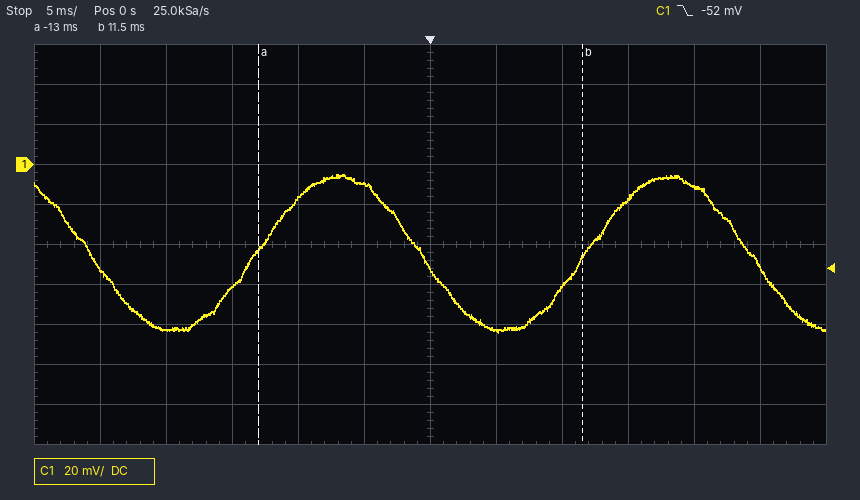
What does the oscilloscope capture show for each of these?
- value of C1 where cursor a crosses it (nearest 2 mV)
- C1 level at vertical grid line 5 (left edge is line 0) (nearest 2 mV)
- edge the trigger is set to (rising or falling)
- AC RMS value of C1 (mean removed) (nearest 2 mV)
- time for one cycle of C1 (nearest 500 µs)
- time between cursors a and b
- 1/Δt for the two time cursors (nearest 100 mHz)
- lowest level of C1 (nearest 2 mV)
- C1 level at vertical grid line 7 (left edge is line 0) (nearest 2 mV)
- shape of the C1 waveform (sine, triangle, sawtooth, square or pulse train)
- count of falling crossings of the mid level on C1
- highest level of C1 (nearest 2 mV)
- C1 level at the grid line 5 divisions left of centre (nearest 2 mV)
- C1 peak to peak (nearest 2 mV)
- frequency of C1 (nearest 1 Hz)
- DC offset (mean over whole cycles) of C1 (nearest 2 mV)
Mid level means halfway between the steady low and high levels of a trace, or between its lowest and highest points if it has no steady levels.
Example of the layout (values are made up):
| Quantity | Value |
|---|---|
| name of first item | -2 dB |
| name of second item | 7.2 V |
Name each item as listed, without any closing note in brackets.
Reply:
| Quantity | Value |
|---|---|
| value of C1 where cursor a crosses it | -42 mV |
| C1 level at vertical grid line 5 (left edge is line 0) | -10 mV |
| edge the trigger is set to | falling |
| AC RMS value of C1 (mean removed) | 28 mV |
| time for one cycle of C1 | 25.0 ms |
| time between cursors a and b | 24.5 ms |
| 1/Δt for the two time cursors | 40.8 Hz |
| lowest level of C1 | -84 mV |
| C1 level at vertical grid line 7 (left edge is line 0) | -84 mV |
| shape of the C1 waveform | sine |
| count of falling crossings of the mid level on C1 | 3 |
| highest level of C1 | -4 mV |
| C1 level at the grid line 5 divisions left of centre | -52 mV |
| C1 peak to peak | 80 mV |
| frequency of C1 | 40 Hz |
| DC offset (mean over whole cycles) of C1 | -44 mV |
